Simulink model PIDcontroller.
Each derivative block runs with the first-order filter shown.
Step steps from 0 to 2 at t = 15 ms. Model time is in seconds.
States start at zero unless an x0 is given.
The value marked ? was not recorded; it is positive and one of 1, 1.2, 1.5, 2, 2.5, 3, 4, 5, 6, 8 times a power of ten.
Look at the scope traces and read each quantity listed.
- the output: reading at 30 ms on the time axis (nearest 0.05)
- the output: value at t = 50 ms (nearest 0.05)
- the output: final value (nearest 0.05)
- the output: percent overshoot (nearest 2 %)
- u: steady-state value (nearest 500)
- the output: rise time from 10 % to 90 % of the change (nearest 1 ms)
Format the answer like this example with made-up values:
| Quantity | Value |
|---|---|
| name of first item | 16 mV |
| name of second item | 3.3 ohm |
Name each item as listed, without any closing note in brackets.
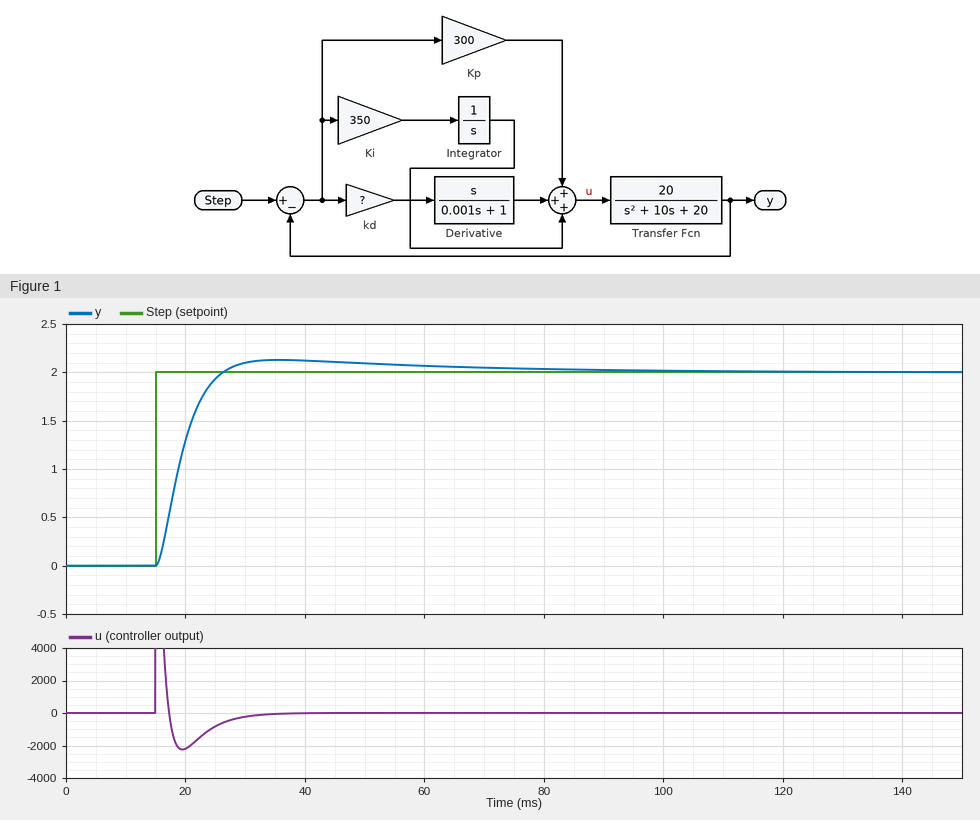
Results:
| Quantity | Value |
|---|---|
| the output: reading at 30 ms on the time axis | 2.10 |
| the output: value at t = 50 ms | 2.10 |
| the output: final value | 2.00 |
| the output: percent overshoot | 6 % |
| u: steady-state value | 0 |
| the output: rise time from 10 % to 90 % of the change | 7 ms |
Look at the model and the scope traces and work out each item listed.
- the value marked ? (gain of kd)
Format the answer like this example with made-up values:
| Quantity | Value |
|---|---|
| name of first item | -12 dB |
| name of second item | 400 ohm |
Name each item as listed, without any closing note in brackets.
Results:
| Quantity | Value |
|---|---|
| the value marked ? | 10 |
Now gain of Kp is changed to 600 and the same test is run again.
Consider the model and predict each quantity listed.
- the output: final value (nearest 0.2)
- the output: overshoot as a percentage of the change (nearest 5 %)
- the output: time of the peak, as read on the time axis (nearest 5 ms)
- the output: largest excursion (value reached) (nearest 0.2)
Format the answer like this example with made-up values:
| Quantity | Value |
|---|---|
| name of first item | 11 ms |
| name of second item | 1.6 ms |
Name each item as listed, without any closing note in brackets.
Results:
| Quantity | Value |
|---|---|
| the output: final value | 2.0 |
| the output: overshoot as a percentage of the change | 15 % |
| the output: time of the peak, as read on the time axis | 30 ms |
| the output: largest excursion (value reached) | 2.2 |
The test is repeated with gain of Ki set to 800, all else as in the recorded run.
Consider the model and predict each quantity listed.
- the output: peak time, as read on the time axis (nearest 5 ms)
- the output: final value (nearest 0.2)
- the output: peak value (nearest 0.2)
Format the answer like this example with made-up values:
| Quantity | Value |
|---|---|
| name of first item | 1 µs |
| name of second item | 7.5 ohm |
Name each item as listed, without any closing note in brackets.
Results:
| Quantity | Value |
|---|---|
| the output: peak time, as read on the time axis | 35 ms |
| the output: final value | 2.0 |
| the output: peak value | 2.2 |
